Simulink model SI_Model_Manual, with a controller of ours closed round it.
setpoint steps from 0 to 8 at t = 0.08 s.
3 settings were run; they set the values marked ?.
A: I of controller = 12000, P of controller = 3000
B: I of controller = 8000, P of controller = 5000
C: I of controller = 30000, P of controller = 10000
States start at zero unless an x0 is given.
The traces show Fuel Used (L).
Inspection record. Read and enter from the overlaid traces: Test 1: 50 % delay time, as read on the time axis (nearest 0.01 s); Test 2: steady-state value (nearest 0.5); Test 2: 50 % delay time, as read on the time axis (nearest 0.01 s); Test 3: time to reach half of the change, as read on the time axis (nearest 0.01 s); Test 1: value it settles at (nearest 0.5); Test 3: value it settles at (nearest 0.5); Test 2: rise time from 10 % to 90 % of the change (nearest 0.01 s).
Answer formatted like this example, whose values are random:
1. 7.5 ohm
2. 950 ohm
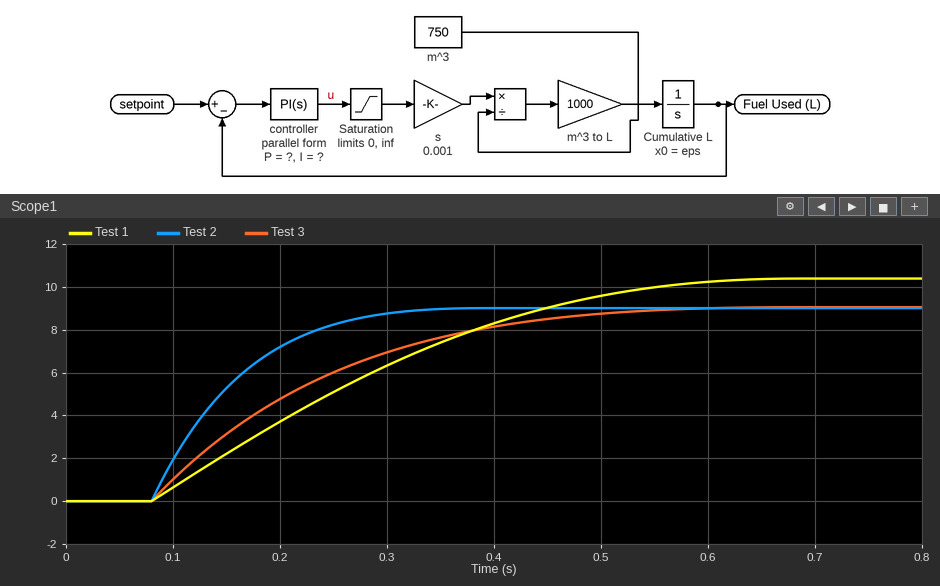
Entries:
1. 0.25 s
2. 9.0
3. 0.14 s
4. 0.19 s
5. 10.5
6. 9.0
7. 0.15 s
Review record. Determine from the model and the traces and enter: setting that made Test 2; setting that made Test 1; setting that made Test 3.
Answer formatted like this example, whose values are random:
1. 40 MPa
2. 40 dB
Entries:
1. C
2. A
3. B
